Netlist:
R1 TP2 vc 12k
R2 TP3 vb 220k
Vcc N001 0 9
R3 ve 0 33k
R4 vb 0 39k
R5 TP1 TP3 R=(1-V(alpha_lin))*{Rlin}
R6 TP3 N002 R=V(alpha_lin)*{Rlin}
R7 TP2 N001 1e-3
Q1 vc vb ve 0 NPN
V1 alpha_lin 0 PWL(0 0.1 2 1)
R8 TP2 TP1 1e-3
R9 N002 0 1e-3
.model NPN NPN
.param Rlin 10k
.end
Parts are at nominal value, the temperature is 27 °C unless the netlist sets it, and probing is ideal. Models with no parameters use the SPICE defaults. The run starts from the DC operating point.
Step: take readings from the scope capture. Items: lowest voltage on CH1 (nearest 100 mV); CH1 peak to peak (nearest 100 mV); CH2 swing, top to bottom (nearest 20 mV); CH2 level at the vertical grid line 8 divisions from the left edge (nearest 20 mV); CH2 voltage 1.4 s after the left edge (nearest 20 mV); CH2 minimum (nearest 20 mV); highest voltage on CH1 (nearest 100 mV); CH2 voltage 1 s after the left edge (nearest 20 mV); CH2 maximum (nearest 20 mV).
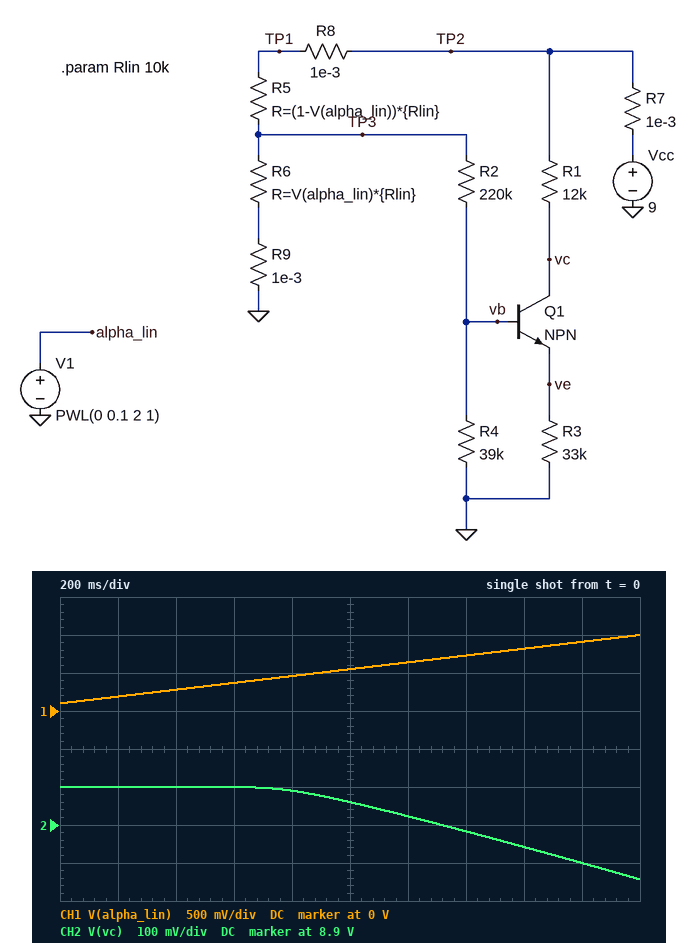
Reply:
100 mV
900 mV
240 mV
8.84 V
8.88 V
8.76 V
1.0 V
8.96 V
9.00 V
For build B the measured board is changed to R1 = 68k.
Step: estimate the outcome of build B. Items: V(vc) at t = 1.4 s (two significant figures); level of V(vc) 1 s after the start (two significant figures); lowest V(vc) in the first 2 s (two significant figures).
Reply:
8.3 V
8.8 V
7.6 V
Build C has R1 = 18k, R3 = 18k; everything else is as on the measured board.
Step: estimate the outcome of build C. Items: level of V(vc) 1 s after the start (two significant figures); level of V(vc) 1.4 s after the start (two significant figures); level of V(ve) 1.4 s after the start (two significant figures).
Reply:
8.9 V
8.7 V
310 mV
